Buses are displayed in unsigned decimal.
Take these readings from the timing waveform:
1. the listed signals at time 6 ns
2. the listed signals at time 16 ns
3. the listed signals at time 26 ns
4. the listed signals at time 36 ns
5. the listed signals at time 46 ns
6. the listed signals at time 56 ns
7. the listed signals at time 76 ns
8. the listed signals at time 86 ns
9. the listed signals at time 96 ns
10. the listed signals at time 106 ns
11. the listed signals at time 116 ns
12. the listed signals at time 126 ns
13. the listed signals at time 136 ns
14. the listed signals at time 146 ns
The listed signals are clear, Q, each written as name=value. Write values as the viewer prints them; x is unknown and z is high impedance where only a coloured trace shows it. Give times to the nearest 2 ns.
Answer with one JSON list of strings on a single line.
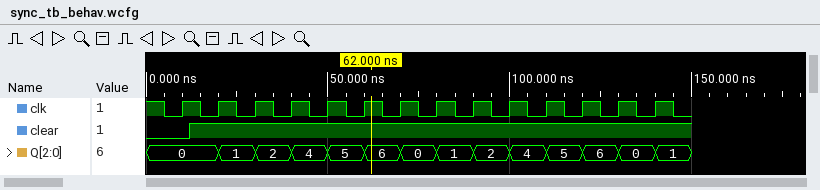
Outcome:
["clear=0, Q=0", "clear=1, Q=0", "clear=1, Q=1", "clear=1, Q=2", "clear=1, Q=4", "clear=1, Q=5", "clear=1, Q=0", "clear=1, Q=1", "clear=1, Q=2", "clear=1, Q=4", "clear=1, Q=5", "clear=1, Q=6", "clear=1, Q=0", "clear=1, Q=1"]
